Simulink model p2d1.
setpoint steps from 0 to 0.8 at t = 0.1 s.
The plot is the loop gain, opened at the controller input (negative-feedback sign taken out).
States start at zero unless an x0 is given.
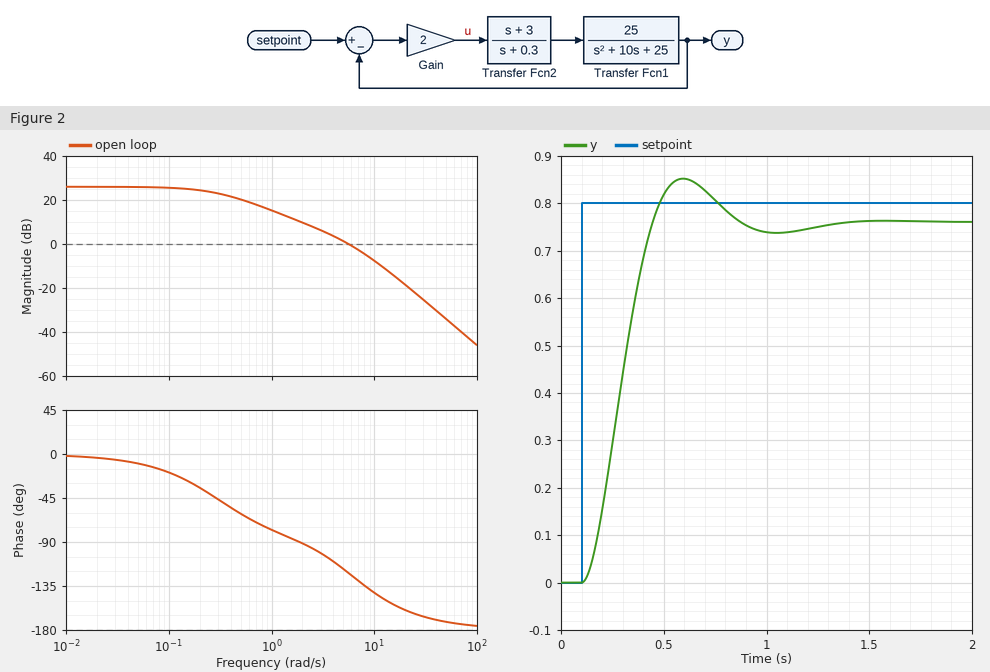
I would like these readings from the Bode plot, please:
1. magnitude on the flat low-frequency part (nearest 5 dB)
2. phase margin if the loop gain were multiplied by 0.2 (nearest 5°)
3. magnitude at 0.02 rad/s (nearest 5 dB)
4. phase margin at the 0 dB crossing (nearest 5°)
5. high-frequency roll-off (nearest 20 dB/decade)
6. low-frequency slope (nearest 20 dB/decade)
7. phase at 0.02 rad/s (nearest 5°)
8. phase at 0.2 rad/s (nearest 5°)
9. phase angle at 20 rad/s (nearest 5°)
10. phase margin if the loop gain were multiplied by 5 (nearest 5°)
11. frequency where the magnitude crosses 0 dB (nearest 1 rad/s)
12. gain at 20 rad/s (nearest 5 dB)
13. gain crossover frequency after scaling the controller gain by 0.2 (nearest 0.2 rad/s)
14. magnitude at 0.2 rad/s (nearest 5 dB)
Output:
25 dB
100°
25 dB
60°
-40 dB/decade
0 dB/decade
-5°
-35°
-160°
25°
6 rad/s
-20 dB
1.2 rad/s
25 dB
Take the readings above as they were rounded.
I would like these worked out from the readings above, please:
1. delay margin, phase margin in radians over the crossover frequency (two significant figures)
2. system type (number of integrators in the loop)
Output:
0.17 s
0
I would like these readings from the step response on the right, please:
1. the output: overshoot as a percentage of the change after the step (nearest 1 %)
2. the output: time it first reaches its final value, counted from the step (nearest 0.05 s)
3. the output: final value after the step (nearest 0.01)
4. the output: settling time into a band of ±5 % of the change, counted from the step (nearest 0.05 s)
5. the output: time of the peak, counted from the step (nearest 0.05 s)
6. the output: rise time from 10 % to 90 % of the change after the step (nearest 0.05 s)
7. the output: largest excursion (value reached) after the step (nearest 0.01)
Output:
12 %
0.35 s
0.76
0.65 s
0.50 s
0.25 s
0.85
